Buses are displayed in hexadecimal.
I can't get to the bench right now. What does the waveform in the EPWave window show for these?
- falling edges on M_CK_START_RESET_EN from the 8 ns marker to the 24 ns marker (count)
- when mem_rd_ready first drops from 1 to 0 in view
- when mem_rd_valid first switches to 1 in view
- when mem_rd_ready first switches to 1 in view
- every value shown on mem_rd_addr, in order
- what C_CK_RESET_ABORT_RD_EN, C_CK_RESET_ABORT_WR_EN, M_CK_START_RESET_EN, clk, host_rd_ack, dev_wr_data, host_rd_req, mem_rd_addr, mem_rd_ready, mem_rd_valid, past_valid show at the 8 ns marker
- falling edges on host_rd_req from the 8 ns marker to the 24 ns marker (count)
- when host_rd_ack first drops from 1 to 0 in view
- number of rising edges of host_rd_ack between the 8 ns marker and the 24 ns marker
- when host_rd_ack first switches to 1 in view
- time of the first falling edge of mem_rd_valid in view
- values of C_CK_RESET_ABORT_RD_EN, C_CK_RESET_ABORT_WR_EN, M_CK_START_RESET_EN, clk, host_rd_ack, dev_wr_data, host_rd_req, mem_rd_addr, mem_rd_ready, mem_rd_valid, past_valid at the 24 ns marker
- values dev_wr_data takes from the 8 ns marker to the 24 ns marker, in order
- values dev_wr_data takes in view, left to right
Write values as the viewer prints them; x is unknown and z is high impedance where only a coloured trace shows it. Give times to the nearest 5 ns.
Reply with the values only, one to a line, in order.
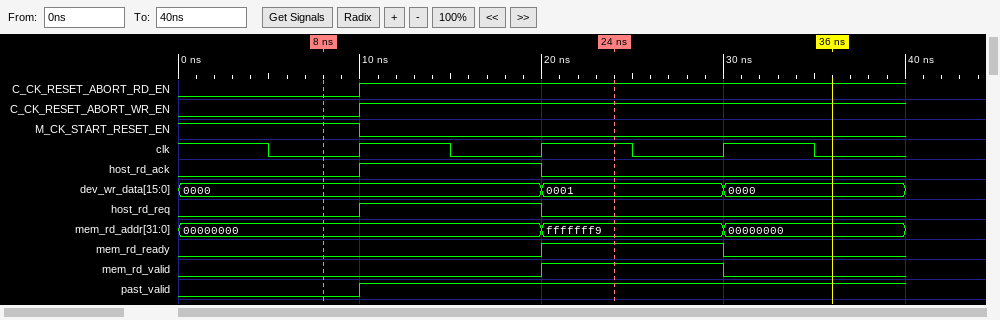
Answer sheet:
1
30 ns
20 ns
20 ns
00000000, fffffff9, 00000000
C_CK_RESET_ABORT_RD_EN=0, C_CK_RESET_ABORT_WR_EN=0, M_CK_START_RESET_EN=1, clk=0, host_rd_ack=0, dev_wr_data=0000, host_rd_req=0, mem_rd_addr=00000000, mem_rd_ready=0, mem_rd_valid=0, past_valid=0
1
20 ns
1
10 ns
30 ns
C_CK_RESET_ABORT_RD_EN=1, C_CK_RESET_ABORT_WR_EN=1, M_CK_START_RESET_EN=0, clk=1, host_rd_ack=0, dev_wr_data=0001, host_rd_req=0, mem_rd_addr=fffffff9, mem_rd_ready=1, mem_rd_valid=1, past_valid=1
0000, 0001
0000, 0001, 0000
